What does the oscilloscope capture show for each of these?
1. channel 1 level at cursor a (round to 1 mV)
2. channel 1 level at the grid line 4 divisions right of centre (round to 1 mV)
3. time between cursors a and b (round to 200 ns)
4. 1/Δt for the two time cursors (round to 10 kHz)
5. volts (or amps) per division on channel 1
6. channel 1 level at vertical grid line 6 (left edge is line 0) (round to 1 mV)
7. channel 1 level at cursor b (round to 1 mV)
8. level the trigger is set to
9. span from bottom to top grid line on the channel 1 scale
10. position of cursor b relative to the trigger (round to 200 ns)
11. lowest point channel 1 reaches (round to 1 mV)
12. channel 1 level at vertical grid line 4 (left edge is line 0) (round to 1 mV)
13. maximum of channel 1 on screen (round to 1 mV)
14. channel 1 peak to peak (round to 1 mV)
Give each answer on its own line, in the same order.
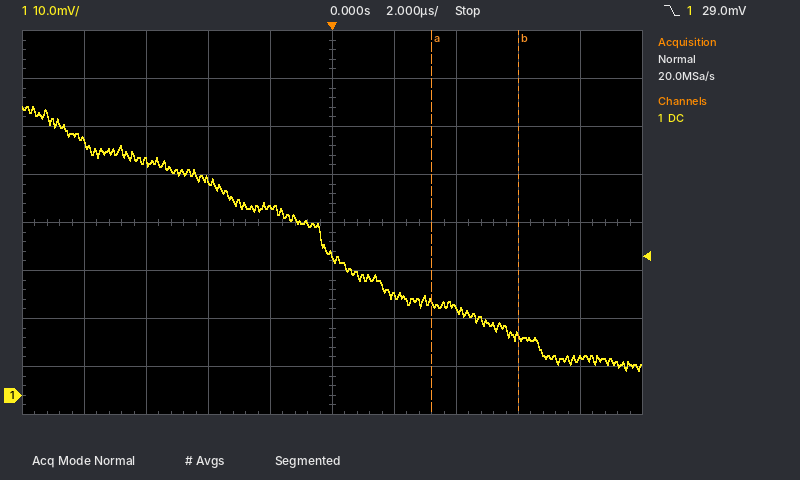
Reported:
19 mV
8 mV
2.8 µs
360 kHz
10 mV
21 mV
12 mV
29.0 mV
80 mV
+6.0 µs
5 mV
39 mV
60 mV
55 mV
